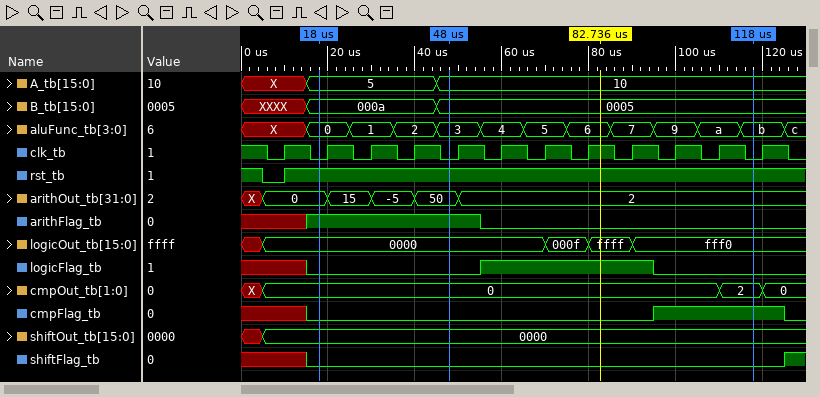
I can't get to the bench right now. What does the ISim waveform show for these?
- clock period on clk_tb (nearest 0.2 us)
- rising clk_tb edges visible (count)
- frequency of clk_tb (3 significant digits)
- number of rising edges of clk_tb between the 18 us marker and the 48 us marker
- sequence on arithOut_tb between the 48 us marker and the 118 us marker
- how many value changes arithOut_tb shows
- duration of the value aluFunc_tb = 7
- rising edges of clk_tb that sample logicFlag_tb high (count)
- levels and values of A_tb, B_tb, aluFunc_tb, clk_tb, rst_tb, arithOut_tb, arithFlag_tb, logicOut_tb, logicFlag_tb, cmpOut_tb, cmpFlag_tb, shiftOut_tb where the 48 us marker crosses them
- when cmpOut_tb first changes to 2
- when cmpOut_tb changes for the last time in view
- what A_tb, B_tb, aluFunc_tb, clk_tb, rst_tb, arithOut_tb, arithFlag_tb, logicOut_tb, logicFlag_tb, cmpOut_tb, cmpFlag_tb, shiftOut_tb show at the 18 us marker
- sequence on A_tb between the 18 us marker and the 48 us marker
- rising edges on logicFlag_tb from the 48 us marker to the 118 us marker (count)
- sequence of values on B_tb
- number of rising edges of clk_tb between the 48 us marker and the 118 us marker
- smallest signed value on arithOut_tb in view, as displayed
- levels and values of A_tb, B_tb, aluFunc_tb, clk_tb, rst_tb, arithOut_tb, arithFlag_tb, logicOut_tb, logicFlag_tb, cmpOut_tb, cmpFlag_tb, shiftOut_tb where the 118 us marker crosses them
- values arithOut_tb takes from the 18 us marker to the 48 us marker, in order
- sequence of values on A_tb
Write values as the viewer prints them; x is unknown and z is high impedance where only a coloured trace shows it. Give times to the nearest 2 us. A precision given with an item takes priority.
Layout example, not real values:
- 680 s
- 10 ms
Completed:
- 10 us
- 12
- 100 kHz
- 3
- 50, 2
- 5
- 10 us
- 4
- A_tb=10, B_tb=0005, aluFunc_tb=3, clk_tb=0, rst_tb=1, arithOut_tb=50, arithFlag_tb=1, logicOut_tb=0000, logicFlag_tb=0, cmpOut_tb=0, cmpFlag_tb=0, shiftOut_tb=0000
- 110 us
- 120 us
- A_tb=5, B_tb=000a, aluFunc_tb=0, clk_tb=0, rst_tb=1, arithOut_tb=0, arithFlag_tb=1, logicOut_tb=0000, logicFlag_tb=0, cmpOut_tb=0, cmpFlag_tb=0, shiftOut_tb=0000
- 5, 10
- 1
- XXXX, 000a, 0005
- 7
- -5
- A_tb=10, B_tb=0005, aluFunc_tb=b, clk_tb=0, rst_tb=1, arithOut_tb=2, arithFlag_tb=0, logicOut_tb=fff0, logicFlag_tb=0, cmpOut_tb=2, cmpFlag_tb=1, shiftOut_tb=0000
- 0, 15, -5, 50
- X, 5, 10
